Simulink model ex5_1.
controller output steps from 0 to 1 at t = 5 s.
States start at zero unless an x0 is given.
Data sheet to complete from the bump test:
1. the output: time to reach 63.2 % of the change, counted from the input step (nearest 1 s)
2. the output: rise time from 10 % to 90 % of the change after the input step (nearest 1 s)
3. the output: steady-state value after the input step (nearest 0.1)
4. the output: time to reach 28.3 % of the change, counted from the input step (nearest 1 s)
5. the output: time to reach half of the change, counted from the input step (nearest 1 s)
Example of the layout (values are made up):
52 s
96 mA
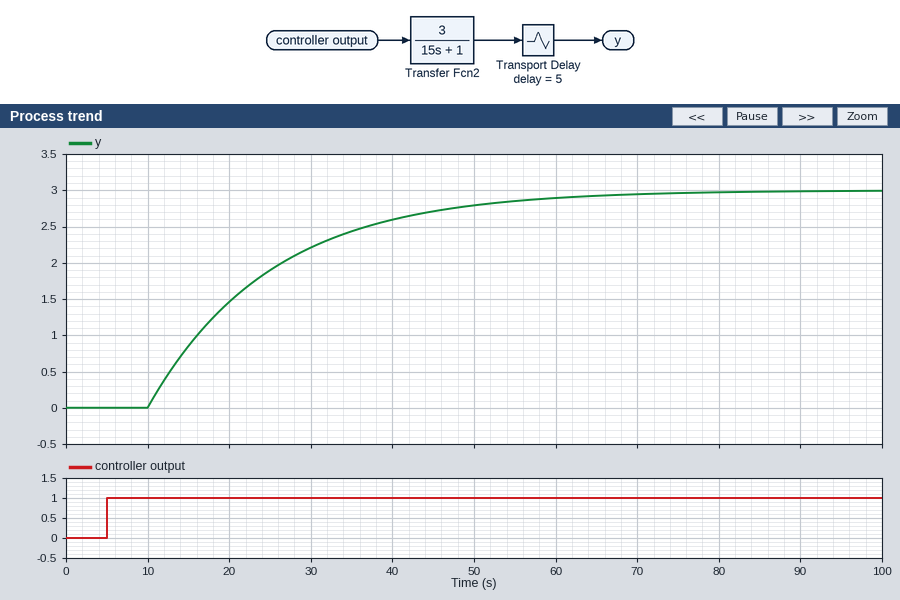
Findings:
20 s
33 s
3.0
10 s
15 s
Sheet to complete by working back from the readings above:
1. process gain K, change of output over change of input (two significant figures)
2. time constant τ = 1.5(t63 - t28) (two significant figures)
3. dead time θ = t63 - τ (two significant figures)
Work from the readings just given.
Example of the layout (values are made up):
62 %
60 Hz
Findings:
3.0
15 s
5.0 s
